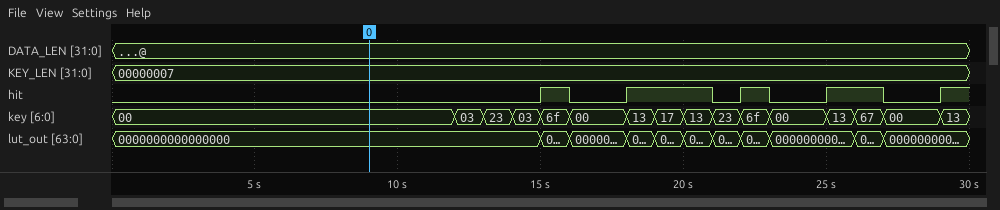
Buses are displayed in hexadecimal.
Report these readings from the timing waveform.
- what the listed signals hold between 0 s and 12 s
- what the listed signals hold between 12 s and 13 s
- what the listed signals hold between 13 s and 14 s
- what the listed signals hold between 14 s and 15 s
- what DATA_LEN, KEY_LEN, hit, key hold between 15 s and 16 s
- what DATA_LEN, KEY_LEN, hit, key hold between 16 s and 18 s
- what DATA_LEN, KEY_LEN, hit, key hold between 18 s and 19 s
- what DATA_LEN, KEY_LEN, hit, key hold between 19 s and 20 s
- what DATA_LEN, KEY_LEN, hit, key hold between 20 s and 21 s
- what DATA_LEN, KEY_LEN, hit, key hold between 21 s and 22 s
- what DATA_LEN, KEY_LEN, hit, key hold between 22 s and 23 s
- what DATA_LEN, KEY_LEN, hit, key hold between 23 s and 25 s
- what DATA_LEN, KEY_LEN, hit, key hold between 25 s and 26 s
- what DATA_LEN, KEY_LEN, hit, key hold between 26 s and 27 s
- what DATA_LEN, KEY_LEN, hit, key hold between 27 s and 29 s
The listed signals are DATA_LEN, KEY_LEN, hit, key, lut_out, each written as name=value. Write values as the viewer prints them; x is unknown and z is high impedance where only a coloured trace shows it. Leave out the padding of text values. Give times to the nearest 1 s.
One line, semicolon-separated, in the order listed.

DATA_LEN=@, KEY_LEN=00000007, hit=0, key=00, lut_out=0000000000000000; DATA_LEN=@, KEY_LEN=00000007, hit=0, key=03, lut_out=0000000000000000; DATA_LEN=@, KEY_LEN=00000007, hit=0, key=23, lut_out=0000000000000000; DATA_LEN=@, KEY_LEN=00000007, hit=0, key=03, lut_out=0000000000000000; DATA_LEN=@, KEY_LEN=00000007, hit=1, key=6f; DATA_LEN=@, KEY_LEN=00000007, hit=0, key=00; DATA_LEN=@, KEY_LEN=00000007, hit=1, key=13; DATA_LEN=@, KEY_LEN=00000007, hit=1, key=17; DATA_LEN=@, KEY_LEN=00000007, hit=1, key=13; DATA_LEN=@, KEY_LEN=00000007, hit=0, key=23; DATA_LEN=@, KEY_LEN=00000007, hit=1, key=6f; DATA_LEN=@, KEY_LEN=00000007, hit=0, key=00; DATA_LEN=@, KEY_LEN=00000007, hit=1, key=13; DATA_LEN=@, KEY_LEN=00000007, hit=1, key=67; DATA_LEN=@, KEY_LEN=00000007, hit=0, key=00
